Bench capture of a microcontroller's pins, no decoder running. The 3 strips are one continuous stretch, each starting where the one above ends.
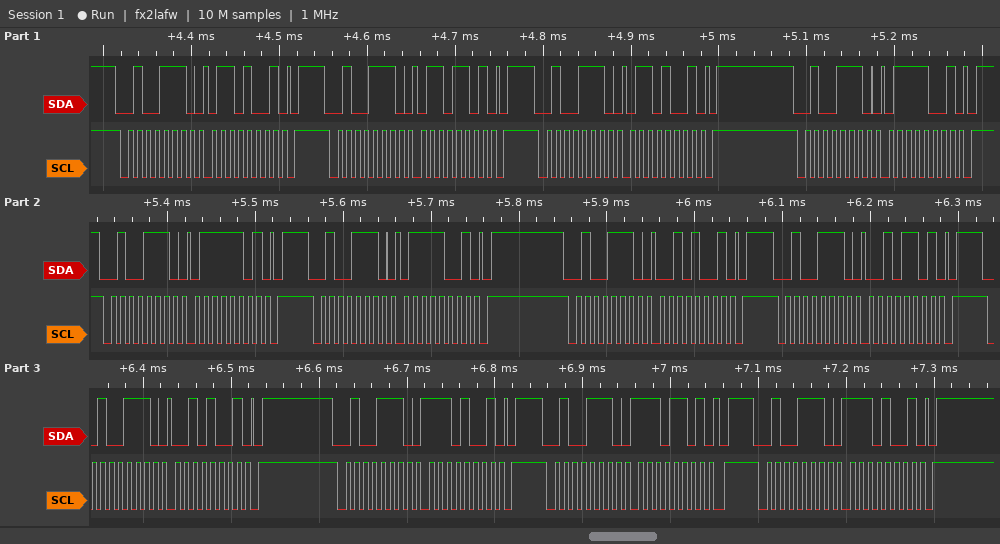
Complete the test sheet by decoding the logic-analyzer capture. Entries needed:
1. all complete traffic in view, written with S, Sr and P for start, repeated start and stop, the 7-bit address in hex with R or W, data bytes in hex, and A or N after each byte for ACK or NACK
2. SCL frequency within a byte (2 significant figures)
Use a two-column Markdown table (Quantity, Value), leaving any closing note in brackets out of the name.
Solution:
| Quantity | Value |
|---|---|
| all complete traffic in view, written with S, Sr and P for start, repeated start and stop, the 7-bit address in hex with R or W, data bytes in hex, and A or N after each byte for ACK or NACK | S 27W A 69 A P S 27W A 6D A P S 27W A 69 A P S 27W A 79 A P S 27W A 7D A P S 27W A 79 A P S 27W A 29 A P S 27W A 2D A P S 27W A 29 A P S 27W A E9 A P S 27W A ED A P S 27W A E9 A P |
| SCL frequency within a byte | 100 kHz |
